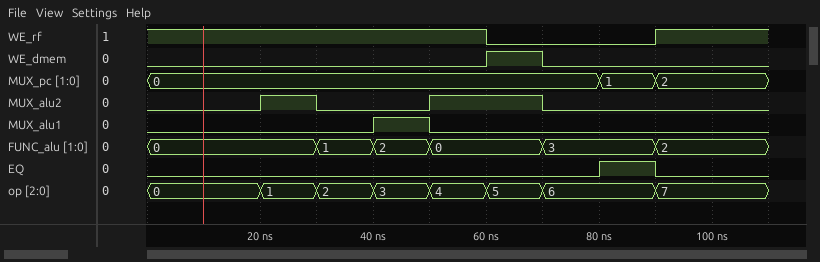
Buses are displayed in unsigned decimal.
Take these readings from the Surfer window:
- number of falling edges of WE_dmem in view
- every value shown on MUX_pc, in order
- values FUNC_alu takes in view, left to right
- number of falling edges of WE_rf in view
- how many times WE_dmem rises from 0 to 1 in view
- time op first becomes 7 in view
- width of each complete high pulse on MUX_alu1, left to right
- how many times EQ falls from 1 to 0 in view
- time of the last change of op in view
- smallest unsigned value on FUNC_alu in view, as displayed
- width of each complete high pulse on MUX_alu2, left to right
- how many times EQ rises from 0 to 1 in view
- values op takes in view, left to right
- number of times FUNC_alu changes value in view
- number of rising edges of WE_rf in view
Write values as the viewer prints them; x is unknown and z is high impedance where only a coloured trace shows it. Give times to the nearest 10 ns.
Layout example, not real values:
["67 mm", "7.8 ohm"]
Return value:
["1", "0, 1, 2", "0, 1, 2, 0, 3, 2", "1", "1", "90 ns", "10 ns", "1", "90 ns", "0", "10 ns, 20 ns", "1", "0, 1, 2, 3, 4, 5, 6, 7", "5", "1"]
